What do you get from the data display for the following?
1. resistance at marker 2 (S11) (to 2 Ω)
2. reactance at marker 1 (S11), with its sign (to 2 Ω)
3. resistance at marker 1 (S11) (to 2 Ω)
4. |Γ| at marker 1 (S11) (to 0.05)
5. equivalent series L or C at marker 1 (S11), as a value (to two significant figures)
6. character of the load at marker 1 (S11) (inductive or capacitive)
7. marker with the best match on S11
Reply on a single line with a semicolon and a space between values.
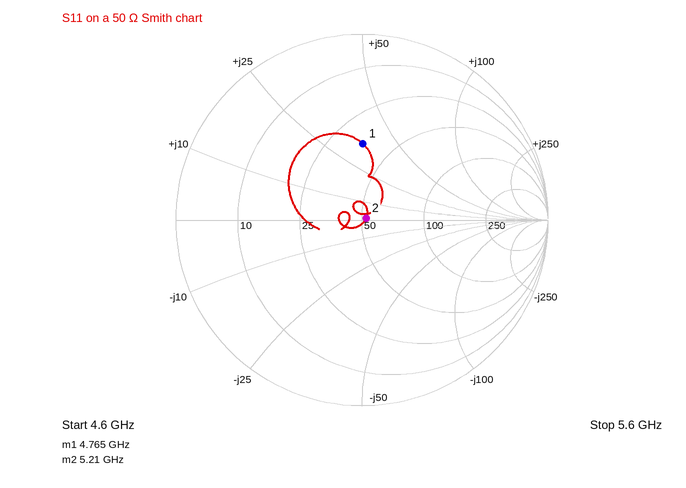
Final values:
52 Ω; +36 Ω; 36 Ω; 0.40; 1.2 nH; inductive; marker 2
